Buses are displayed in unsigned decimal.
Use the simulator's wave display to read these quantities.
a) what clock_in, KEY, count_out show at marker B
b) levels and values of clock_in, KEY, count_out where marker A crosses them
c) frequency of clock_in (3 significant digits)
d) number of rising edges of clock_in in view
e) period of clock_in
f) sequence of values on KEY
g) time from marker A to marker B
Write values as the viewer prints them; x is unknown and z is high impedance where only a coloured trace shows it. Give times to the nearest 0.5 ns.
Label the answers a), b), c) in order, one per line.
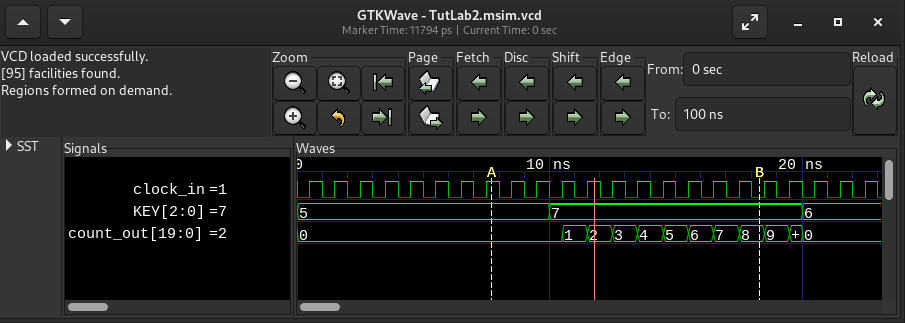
a) clock_in=0, KEY=7, count_out=8
b) clock_in=1, KEY=5, count_out=0
c) 1.00 GHz
d) 23
e) 1 ns
f) 5, 7, 6
g) 10.5 ns
